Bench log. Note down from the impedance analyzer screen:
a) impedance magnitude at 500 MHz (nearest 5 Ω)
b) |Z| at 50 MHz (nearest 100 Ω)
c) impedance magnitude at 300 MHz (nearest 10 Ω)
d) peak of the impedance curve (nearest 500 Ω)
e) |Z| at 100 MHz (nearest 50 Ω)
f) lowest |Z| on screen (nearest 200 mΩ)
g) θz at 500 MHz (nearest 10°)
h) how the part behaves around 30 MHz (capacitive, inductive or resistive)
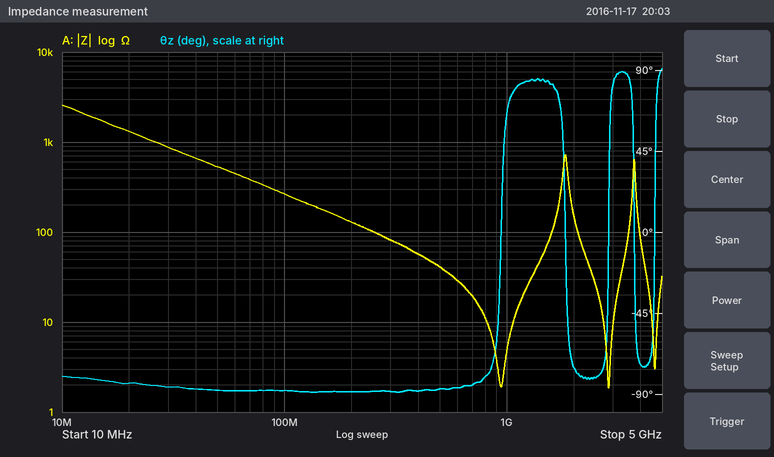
40 Ω
500 Ω
80 Ω
2.5 kΩ
250 Ω
1.8 Ω
-90°
capacitive
